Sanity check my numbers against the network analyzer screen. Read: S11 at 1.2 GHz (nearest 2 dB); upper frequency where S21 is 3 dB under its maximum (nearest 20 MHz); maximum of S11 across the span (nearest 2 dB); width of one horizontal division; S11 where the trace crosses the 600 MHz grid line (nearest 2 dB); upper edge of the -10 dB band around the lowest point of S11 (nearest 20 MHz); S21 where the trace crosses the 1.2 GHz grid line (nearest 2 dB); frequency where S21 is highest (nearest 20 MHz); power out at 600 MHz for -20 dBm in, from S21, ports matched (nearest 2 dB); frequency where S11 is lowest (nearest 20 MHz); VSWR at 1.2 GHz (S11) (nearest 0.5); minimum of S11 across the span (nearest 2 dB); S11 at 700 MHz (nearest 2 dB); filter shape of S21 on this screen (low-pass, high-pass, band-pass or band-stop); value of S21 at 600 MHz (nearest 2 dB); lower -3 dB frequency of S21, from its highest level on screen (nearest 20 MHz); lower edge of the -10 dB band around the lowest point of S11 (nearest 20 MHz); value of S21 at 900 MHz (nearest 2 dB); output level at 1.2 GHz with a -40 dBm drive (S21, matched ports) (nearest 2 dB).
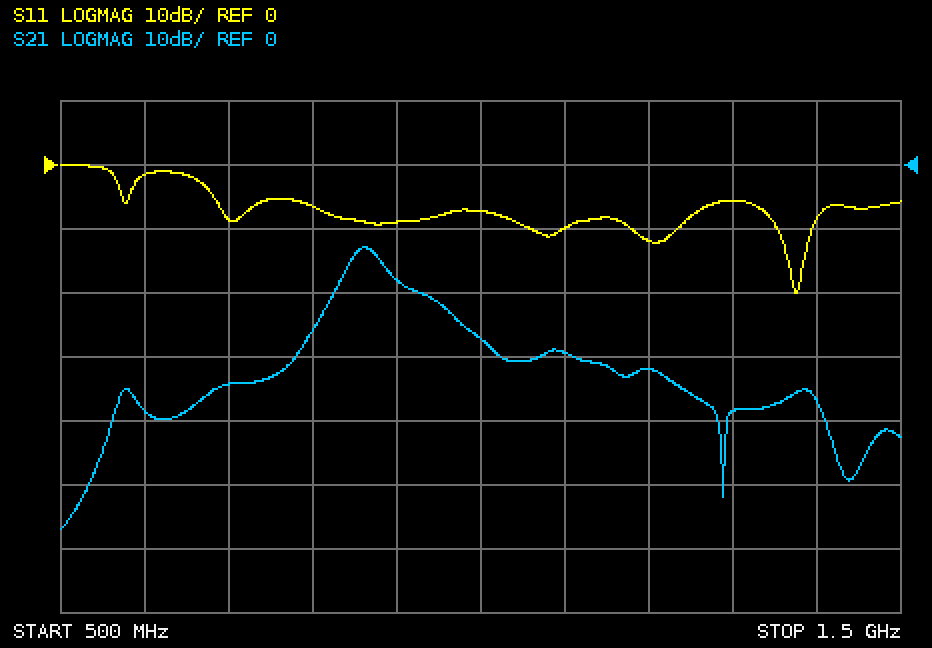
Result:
-12 dB
880 MHz
0 dB
100 MHz
-2 dB
1.40 GHz
-32 dB
860 MHz
-58 dBm
1.38 GHz
1.5
-20 dB
-8 dB
band-pass
-38 dB
840 MHz
1.36 GHz
-18 dB
-72 dBm
